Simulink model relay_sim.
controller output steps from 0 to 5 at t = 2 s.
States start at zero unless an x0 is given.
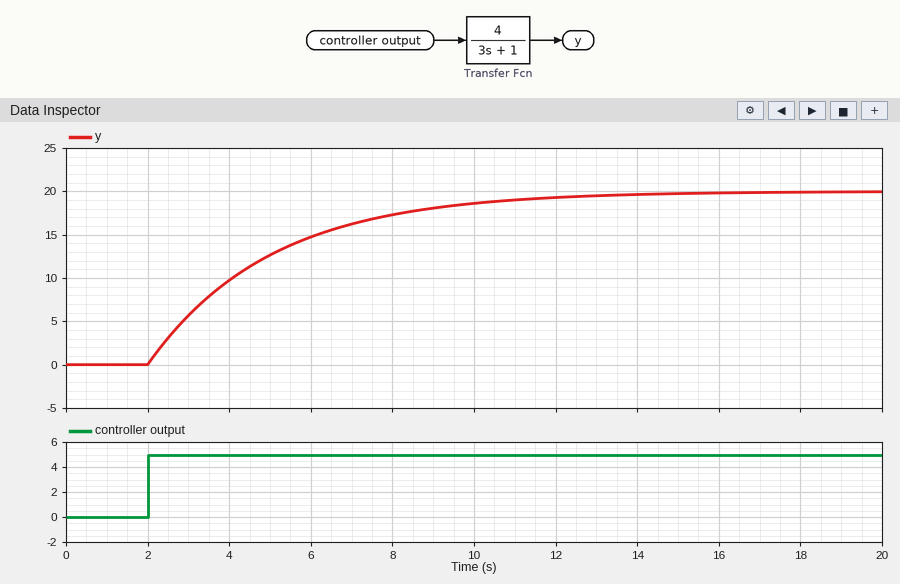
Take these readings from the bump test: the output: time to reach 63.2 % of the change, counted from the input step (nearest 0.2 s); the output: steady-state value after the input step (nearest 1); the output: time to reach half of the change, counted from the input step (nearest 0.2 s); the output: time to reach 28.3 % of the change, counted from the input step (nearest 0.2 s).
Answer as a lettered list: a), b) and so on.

a) 3.0 s
b) 20
c) 2.0 s
d) 1.0 s
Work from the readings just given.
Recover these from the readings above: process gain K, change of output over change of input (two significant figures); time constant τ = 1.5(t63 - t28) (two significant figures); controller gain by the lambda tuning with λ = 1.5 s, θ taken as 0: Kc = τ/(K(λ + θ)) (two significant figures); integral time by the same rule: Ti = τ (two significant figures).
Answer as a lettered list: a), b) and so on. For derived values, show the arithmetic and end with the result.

a) (20 - 0) / 5 = 4.0
b) 1.5 × (3 - 1) = 3.0 s
c) 3 / (4 × (1.5 + 0)) = 0.50
d) 3.0 s
